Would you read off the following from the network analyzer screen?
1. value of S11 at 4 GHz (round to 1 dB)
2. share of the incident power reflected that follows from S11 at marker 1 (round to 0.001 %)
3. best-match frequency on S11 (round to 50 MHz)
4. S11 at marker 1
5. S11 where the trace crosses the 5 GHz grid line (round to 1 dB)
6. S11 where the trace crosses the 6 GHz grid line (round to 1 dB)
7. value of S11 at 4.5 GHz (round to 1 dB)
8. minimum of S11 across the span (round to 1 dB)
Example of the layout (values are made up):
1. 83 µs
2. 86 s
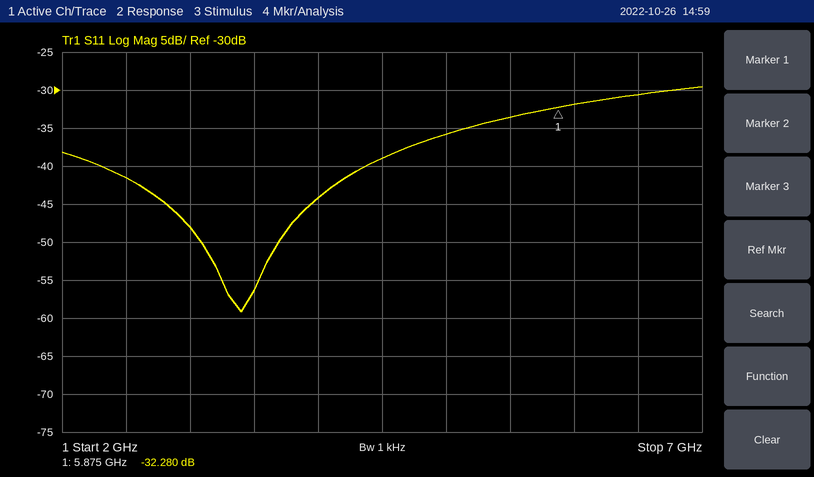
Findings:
1. -44 dB
2. 0.059 %
3. 3.40 GHz
4. -32.280 dB
5. -36 dB
6. -32 dB
7. -39 dB
8. -59 dB
